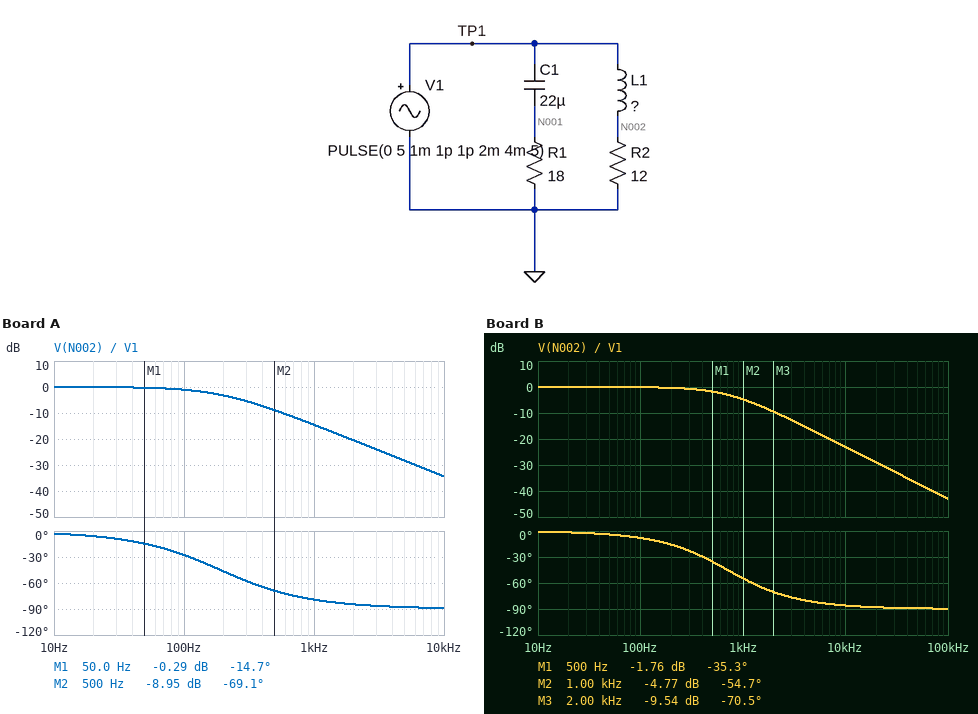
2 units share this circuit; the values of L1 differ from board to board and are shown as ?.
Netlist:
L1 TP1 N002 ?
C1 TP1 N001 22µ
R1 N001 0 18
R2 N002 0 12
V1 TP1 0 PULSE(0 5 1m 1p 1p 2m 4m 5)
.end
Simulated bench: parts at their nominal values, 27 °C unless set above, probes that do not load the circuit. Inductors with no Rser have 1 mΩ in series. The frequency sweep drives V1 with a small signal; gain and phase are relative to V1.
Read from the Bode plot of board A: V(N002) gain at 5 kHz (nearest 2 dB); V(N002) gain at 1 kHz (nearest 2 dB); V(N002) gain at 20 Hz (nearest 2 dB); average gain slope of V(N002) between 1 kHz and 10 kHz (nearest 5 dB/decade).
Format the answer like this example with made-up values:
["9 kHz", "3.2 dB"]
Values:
["-28 dB", "-14 dB", "0 dB", "-20 dB/decade"]
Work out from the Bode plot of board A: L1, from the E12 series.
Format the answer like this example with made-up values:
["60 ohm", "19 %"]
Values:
["10 mH"]
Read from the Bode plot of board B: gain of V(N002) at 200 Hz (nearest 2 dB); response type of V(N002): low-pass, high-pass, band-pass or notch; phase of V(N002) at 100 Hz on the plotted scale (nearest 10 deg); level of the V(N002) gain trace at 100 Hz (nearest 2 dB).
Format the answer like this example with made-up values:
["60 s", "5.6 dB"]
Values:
["0 dB", "low-pass", "-10 deg", "0 dB"]
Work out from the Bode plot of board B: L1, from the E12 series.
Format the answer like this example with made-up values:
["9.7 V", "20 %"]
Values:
["2.7 mH"]
